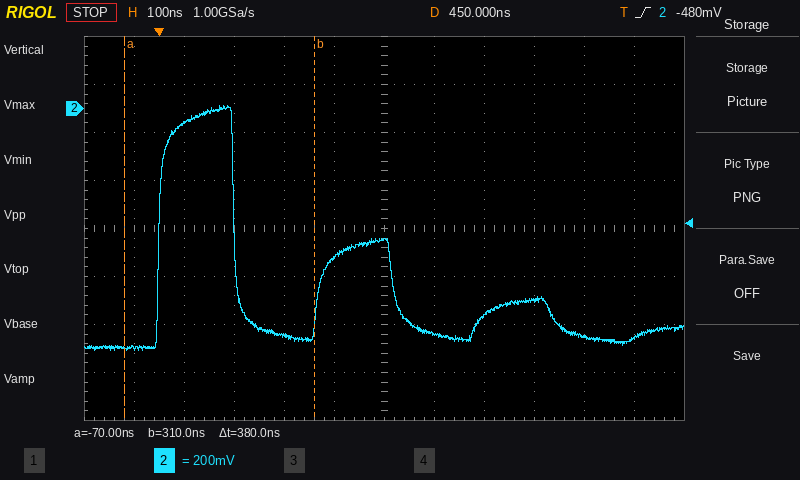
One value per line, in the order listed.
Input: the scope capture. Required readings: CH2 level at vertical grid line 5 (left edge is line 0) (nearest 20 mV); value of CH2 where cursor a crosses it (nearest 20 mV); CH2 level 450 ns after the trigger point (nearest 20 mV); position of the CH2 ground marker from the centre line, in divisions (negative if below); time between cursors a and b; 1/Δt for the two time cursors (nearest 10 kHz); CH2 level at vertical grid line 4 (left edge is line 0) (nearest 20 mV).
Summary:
-620 mV
-1.00 V
-540 mV
+2.5 div
380 ns
2.63 MHz
-940 mV
